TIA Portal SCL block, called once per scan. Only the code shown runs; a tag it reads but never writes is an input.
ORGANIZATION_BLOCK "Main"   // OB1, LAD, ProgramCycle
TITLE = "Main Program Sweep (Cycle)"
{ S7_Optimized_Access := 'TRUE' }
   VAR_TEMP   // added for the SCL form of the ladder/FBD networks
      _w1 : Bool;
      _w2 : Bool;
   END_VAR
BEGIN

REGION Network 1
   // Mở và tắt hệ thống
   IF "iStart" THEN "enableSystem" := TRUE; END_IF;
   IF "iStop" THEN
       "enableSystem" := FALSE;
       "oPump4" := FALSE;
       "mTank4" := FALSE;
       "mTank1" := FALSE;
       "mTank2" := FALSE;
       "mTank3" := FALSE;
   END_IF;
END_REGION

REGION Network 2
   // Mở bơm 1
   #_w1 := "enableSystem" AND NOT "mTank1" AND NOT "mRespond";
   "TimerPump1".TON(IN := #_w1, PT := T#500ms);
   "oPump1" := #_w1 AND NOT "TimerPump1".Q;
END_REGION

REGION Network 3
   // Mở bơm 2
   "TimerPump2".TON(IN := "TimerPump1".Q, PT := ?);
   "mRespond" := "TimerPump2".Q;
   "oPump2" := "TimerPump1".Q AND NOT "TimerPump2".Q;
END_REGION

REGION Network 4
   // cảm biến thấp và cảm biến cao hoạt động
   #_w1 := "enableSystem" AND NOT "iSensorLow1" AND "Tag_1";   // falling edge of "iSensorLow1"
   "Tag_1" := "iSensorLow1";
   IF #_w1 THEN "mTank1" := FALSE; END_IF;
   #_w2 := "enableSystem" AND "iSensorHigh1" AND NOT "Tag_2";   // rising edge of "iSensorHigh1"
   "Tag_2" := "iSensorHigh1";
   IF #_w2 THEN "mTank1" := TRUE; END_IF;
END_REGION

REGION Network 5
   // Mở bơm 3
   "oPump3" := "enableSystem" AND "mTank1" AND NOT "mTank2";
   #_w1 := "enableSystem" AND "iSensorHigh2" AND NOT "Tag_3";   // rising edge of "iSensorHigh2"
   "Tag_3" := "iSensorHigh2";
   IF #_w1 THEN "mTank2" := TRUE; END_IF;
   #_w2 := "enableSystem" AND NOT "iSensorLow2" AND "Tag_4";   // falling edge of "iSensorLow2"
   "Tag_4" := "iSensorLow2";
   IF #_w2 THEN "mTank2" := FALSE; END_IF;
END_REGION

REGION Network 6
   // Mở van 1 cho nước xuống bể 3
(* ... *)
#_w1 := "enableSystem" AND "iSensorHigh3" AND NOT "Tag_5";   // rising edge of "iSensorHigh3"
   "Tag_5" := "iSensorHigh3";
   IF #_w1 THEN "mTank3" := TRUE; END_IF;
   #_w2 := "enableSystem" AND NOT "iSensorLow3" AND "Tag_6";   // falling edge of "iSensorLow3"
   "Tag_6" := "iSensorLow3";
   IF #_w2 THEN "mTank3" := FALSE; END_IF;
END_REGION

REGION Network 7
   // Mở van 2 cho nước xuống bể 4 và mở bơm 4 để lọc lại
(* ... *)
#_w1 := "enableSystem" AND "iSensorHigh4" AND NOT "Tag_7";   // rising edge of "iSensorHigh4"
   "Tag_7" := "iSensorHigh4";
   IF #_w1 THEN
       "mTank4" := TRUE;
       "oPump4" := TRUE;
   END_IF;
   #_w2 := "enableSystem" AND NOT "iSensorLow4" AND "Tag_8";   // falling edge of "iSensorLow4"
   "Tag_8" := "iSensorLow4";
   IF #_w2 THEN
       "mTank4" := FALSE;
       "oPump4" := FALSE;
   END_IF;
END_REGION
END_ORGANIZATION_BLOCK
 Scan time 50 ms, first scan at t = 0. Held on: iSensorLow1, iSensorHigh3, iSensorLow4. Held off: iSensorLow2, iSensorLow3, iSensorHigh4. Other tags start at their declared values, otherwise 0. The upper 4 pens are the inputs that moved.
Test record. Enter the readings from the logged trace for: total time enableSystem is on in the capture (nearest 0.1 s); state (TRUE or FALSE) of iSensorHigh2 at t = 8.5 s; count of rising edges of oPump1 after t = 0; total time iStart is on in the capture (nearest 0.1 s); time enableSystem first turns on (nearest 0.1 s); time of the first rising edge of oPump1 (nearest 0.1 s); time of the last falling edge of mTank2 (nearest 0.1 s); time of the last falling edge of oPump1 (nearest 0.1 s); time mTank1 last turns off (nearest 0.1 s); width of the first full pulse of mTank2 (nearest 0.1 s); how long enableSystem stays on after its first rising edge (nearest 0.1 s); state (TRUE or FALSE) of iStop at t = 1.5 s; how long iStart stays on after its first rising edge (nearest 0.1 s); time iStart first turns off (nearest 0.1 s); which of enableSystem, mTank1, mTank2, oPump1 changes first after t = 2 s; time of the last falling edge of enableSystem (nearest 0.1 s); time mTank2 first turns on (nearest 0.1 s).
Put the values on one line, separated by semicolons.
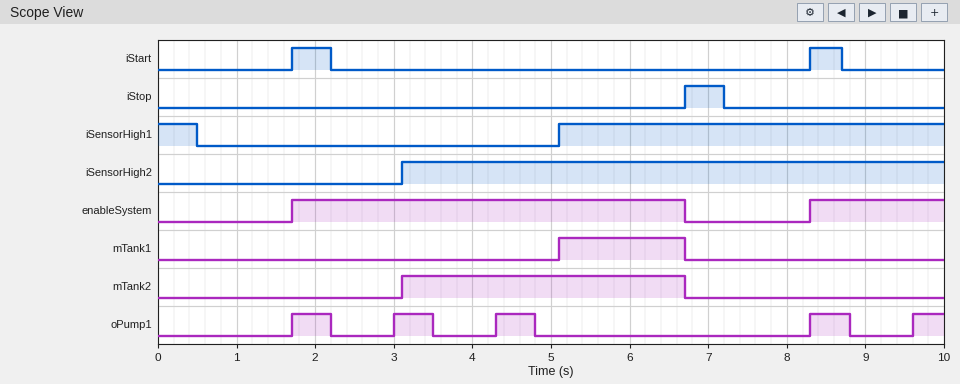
6.7 s; TRUE; 5; 0.9 s; 1.7 s; 1.7 s; 6.7 s; 8.8 s; 6.7 s; 3.6 s; 5.0 s; FALSE; 0.5 s; 2.2 s; oPump1; 6.7 s; 3.1 s
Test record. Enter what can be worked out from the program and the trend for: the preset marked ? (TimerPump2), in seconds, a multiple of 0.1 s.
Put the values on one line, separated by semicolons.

0.7 s
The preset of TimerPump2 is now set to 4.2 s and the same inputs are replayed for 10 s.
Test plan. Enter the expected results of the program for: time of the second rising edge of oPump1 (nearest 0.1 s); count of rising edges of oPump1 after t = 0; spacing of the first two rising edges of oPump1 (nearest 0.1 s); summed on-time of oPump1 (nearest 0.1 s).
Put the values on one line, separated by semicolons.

8.3 s; 2; 6.6 s; 1.0 s
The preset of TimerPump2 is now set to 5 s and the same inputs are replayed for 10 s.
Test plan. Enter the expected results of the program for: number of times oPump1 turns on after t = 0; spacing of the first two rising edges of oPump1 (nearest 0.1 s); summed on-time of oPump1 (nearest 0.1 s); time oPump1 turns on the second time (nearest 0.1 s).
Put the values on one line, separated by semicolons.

2; 6.6 s; 1.0 s; 8.3 s
